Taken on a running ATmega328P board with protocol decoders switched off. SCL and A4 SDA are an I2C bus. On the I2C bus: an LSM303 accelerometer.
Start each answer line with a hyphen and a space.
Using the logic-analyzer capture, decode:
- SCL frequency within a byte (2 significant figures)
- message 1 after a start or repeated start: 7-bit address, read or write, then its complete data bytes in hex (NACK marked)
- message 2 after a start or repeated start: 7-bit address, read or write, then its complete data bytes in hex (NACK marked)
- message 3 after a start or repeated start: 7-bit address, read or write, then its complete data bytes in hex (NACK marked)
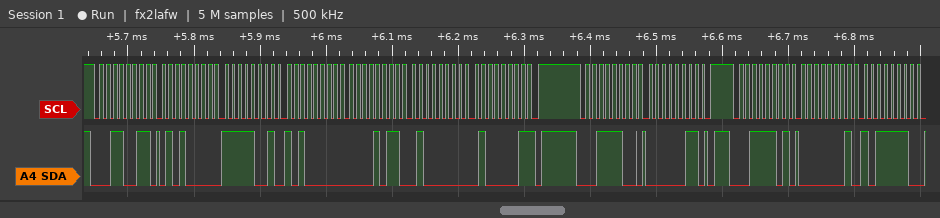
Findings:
- 100 kHz
- 0x19 read: 50 F9 A0 0B 40 41 NACK
- 0x1E write: 03
- 0x1E read: 01 BE
